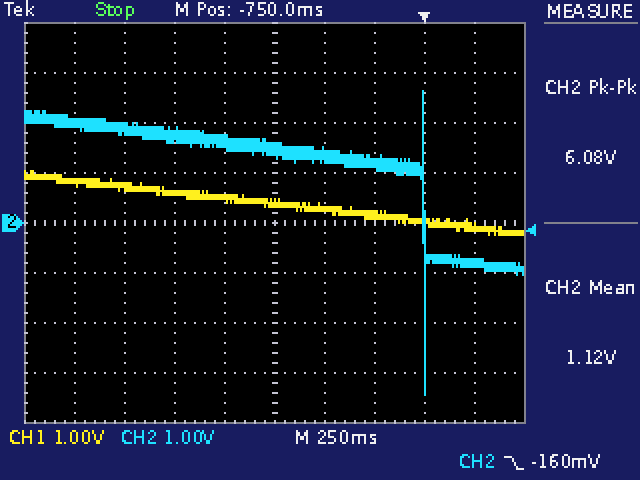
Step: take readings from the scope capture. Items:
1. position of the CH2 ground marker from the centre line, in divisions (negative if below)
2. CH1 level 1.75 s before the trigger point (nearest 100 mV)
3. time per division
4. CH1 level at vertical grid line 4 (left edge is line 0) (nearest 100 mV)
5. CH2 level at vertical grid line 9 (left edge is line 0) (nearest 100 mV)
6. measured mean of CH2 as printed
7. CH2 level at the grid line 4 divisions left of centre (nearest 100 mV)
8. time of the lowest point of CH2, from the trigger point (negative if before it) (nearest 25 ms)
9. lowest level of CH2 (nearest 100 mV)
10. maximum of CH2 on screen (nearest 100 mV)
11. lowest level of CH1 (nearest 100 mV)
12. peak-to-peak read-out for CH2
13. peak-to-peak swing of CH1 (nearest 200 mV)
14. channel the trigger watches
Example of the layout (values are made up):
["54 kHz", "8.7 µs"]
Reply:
["0.0 div", "800 mV", "250 ms", "500 mV", "-800 mV", "1.12 V", "2.0 V", "0 ms", "-3.4 V", "2.6 V", "-200 mV", "6.08 V", "1.2 V", "CH2"]
